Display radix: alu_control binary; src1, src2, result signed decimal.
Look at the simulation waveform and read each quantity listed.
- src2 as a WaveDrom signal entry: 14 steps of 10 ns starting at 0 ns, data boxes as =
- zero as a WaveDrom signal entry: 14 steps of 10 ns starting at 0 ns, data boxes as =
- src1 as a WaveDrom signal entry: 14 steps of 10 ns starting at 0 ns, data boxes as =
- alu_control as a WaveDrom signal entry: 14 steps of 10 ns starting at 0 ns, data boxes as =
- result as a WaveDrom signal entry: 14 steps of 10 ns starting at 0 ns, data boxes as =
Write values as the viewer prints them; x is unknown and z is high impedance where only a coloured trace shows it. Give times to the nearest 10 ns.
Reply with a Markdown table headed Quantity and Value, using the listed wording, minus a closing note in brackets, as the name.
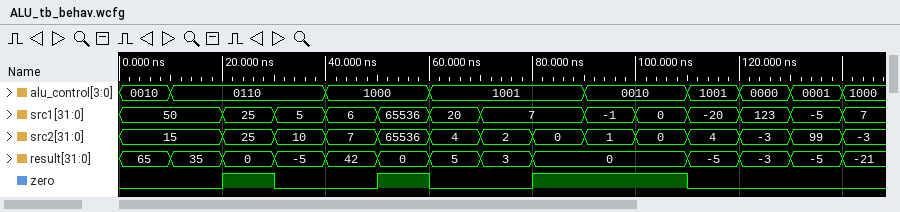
| Quantity | Value |
|---|---|
| src2 as a WaveDrom signal entry: 14 steps of 10 ns starting at 0 ns, data boxes as = | {name: 'src2', wave: '=.============', data: '15 25 10 7 65536 4 2 0 1 0 4 -3 99'} |
| zero as a WaveDrom signal entry: 14 steps of 10 ns starting at 0 ns, data boxes as = | {name: 'zero', wave: '0.10.10.1..0..'} |
| src1 as a WaveDrom signal entry: 14 steps of 10 ns starting at 0 ns, data boxes as = | {name: 'src1', wave: '=.======.=====', data: '50 25 5 6 65536 20 7 -1 0 -20 123 -5'} |
| alu_control as a WaveDrom signal entry: 14 steps of 10 ns starting at 0 ns, data boxes as = | {name: 'alu_control', wave: '==..=.=..=.===', data: '0010 0110 1000 1001 0010 1001 0000 0001'} |
| result as a WaveDrom signal entry: 14 steps of 10 ns starting at 0 ns, data boxes as = | {name: 'result', wave: '=========..===', data: '65 35 0 -5 42 0 5 3 0 -5 -3 -5'} |
